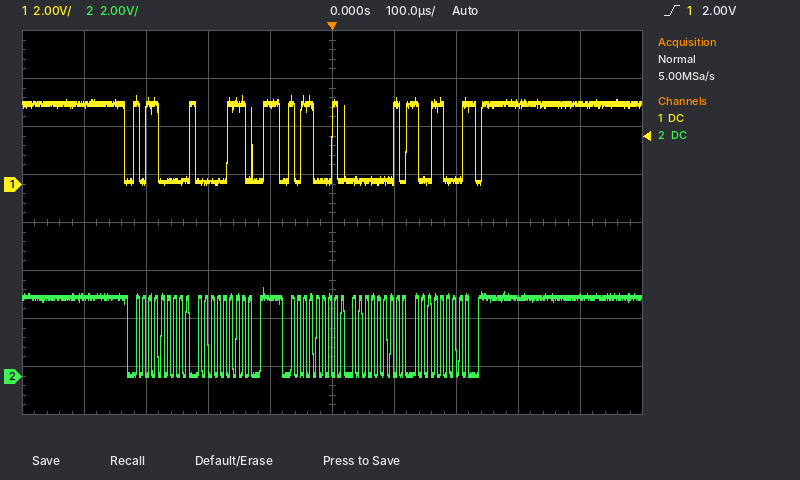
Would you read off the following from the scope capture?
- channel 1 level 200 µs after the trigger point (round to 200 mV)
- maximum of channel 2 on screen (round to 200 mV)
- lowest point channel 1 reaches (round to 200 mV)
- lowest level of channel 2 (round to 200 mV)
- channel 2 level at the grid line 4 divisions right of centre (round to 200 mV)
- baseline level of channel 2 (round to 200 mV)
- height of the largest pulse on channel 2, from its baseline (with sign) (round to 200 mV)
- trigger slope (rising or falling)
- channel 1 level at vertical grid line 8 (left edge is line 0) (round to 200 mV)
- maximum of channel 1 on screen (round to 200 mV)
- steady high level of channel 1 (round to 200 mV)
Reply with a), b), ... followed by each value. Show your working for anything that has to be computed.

a) 200 mV
b) 3.6 V
c) 0.0 V
d) 0.0 V
e) 3.4 V
f) 3.2 V
g) 0.0 V − (3.2 V) = -3.2 V
h) rising
i) 3.4 V
j) 3.6 V
k) 3.4 V
